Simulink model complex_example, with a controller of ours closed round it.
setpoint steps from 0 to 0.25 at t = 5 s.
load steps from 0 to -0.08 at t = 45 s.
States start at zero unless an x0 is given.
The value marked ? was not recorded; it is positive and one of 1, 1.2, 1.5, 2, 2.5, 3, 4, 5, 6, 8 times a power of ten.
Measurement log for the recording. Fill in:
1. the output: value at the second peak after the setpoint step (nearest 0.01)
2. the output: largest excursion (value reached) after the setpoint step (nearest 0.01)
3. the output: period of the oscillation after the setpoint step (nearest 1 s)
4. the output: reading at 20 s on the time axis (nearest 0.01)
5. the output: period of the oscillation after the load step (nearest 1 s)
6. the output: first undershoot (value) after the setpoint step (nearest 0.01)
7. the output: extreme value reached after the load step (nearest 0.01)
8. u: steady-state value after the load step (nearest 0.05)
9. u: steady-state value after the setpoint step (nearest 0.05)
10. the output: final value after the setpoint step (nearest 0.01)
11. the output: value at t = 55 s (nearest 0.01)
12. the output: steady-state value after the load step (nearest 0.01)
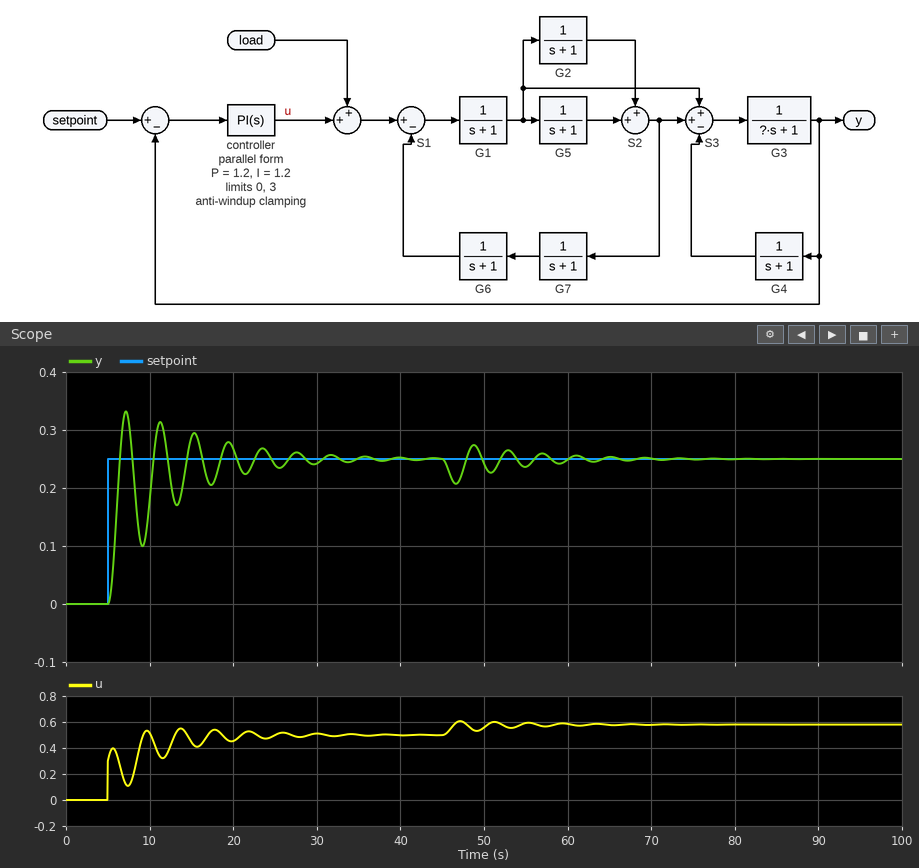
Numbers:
0.31
0.33
4 s
0.27
4 s
0.10
0.21
0.60
0.50
0.25
0.24
0.25
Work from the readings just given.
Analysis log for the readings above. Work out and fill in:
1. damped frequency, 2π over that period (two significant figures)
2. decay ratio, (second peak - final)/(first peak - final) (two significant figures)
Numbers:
1.6 rad/s
0.75
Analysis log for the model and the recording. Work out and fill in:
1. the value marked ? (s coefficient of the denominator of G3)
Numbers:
1
